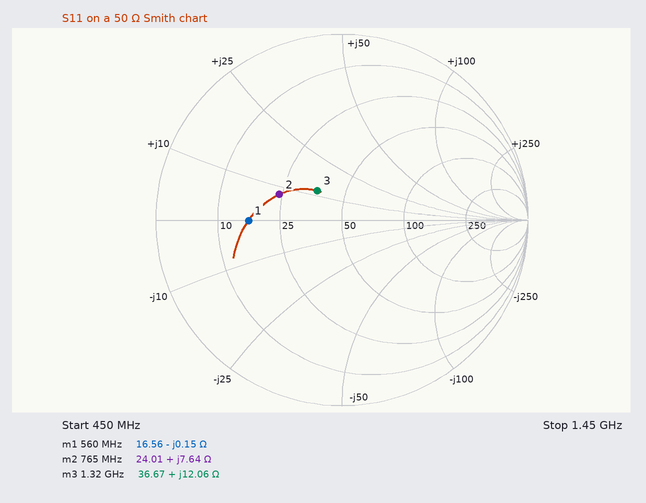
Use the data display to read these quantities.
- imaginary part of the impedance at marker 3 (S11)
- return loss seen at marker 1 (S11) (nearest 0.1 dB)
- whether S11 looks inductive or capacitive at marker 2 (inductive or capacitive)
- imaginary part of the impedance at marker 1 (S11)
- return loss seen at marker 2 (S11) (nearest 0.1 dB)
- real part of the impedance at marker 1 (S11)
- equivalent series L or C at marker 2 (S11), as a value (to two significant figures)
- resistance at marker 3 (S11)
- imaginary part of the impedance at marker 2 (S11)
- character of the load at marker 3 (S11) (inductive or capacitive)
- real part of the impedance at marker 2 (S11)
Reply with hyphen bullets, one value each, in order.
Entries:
- +12.06 Ω
- 6.0 dB
- inductive
- -0.15 Ω
- 8.8 dB
- 16.56 Ω
- 1.6 nH
- 36.67 Ω
- +7.64 Ω
- inductive
- 24.01 Ω
